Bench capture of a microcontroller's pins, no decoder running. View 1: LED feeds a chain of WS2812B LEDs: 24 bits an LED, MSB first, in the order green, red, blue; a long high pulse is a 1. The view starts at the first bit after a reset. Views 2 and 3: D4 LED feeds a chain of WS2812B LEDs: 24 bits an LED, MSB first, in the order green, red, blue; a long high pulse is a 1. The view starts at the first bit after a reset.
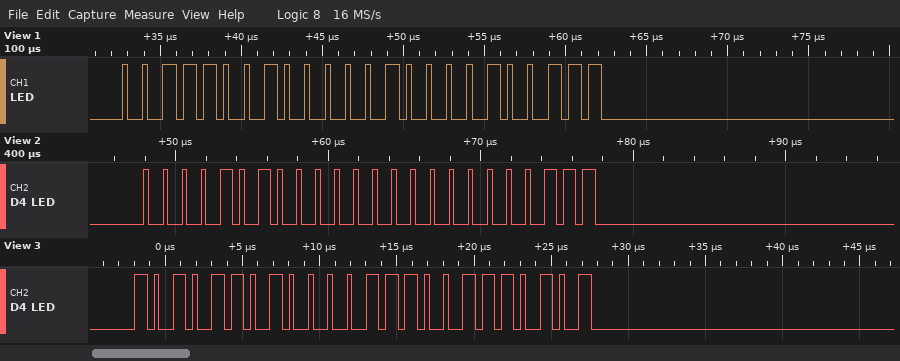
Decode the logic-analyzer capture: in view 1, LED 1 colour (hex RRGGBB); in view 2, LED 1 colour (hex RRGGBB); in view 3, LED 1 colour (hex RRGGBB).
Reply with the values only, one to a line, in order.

#043927
#000A07
#0EAD75
